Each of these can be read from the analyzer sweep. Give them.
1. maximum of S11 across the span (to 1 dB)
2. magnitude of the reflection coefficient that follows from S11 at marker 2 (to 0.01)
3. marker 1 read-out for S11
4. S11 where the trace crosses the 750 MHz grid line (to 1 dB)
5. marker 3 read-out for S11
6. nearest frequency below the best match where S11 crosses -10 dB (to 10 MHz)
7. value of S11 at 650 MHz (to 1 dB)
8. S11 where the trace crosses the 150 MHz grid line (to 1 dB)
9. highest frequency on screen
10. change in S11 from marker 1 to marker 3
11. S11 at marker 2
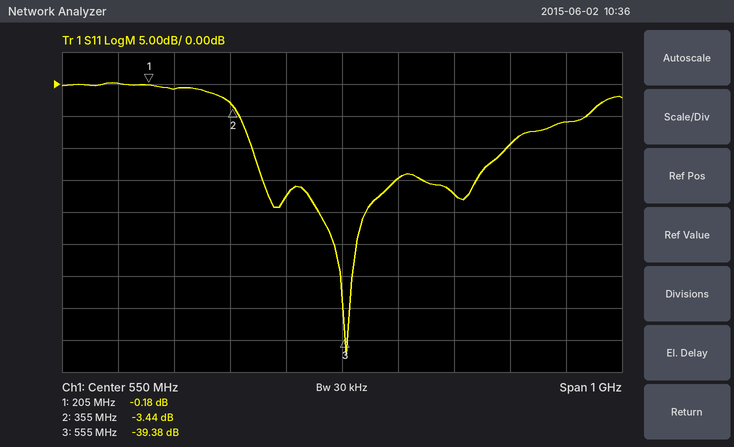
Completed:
0 dB
0.67
-0.18 dB
-17 dB
-39.38 dB
390 MHz
-15 dB
0 dB
1.05 GHz
-39.20 dB
-3.44 dB
